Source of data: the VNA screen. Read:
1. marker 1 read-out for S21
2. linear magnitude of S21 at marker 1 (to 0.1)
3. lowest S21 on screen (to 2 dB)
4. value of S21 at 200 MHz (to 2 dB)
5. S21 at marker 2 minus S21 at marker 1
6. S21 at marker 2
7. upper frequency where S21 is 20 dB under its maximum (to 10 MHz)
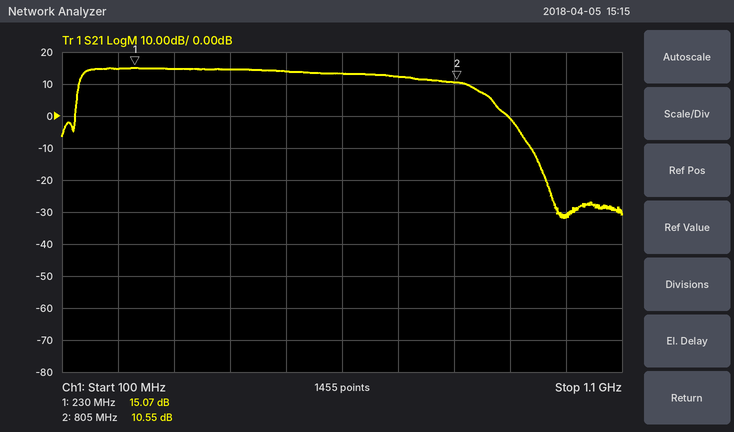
15.07 dB
5.7
-32 dB
14 dB
-4.52 dB
10.55 dB
920 MHz
